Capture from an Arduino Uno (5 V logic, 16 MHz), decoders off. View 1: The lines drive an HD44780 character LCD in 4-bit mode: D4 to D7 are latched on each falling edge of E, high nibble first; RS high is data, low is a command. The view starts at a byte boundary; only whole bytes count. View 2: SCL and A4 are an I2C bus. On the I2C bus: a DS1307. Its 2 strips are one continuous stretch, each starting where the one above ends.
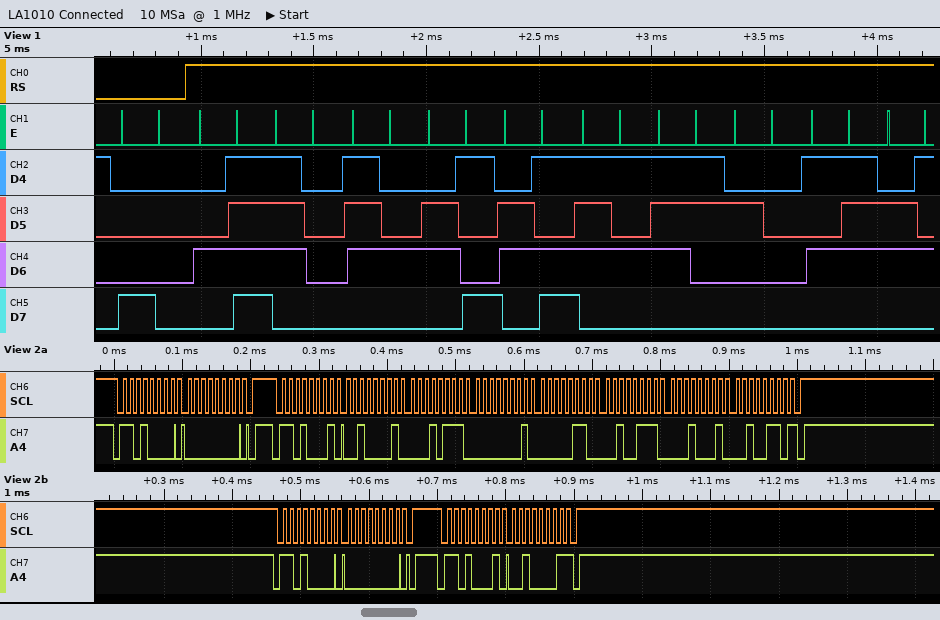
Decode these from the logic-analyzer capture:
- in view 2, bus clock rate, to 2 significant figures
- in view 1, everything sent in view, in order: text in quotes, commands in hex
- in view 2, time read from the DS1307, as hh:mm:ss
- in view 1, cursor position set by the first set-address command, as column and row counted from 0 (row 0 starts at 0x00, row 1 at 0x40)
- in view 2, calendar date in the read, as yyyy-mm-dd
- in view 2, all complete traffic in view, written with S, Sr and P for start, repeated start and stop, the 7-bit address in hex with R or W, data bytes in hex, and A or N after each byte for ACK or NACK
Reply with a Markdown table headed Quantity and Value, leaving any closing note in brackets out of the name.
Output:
| Quantity | Value |
|---|---|
| in view 2, bus clock rate, to 2 significant figures | 100 kHz |
| in view 1, everything sent in view, in order: text in quotes, commands in hex | 0x80 "Optimus We" |
| in view 2, time read from the DS1307, as hh:mm:ss | 01:17:21 |
| in view 1, cursor position set by the first set-address command, as column and row counted from 0 | column 0, row 0 |
| in view 2, calendar date in the read, as yyyy-mm-dd | 2026-11-27 |
| in view 2, all complete traffic in view, written with S, Sr and P for start, repeated start and stop, the 7-bit address in hex with R or W, data bytes in hex, and A or N after each byte for ACK or NACK | S 68W A 00 A P S 68R A 21 A 17 A 01 A 06 A 27 A 11 A 26 N P S 68W A 00 A P S 68R A 21 N P |
